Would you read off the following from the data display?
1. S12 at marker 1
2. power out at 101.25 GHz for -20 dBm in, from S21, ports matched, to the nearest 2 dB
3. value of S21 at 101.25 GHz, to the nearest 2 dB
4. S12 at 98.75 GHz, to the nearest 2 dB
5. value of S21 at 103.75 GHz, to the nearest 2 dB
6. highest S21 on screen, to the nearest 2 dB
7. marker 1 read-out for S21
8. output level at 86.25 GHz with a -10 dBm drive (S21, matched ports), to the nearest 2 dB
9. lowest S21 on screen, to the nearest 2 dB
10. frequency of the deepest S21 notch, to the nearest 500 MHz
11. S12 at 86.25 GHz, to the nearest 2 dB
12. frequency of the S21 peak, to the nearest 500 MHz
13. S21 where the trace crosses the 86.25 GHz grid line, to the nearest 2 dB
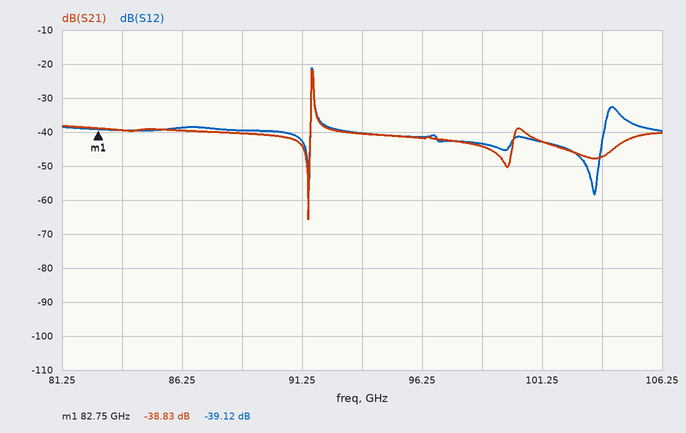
-39.12 dB
-62 dBm
-42 dB
-44 dB
-48 dB
-22 dB
-38.83 dB
-50 dBm
-66 dB
91.5 GHz
-38 dB
91.5 GHz
-40 dB
